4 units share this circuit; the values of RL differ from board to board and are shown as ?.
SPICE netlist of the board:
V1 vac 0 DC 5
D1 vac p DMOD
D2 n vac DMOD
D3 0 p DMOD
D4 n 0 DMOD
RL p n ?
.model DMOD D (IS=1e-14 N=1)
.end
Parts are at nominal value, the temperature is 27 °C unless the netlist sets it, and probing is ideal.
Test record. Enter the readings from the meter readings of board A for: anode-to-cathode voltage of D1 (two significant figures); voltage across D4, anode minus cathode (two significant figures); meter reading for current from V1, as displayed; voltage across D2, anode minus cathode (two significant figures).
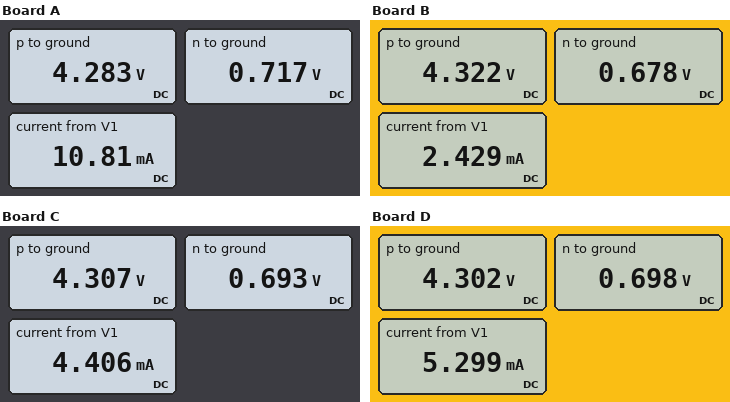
720 mV
720 mV
10.81 mA
-4.3 V
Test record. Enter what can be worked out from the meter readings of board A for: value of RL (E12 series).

330 Ω
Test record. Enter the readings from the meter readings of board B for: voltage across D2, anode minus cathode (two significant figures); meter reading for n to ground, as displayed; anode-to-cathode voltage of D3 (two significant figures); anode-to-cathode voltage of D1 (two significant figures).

-4.3 V
0.678 V
-4.3 V
680 mV
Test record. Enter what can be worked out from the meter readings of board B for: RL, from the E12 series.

1.5 kΩ
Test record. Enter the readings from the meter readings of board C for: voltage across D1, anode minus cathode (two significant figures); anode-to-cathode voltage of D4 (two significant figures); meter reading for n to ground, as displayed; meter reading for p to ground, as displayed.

690 mV
690 mV
0.693 V
4.307 V
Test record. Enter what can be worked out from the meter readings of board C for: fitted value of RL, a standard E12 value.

820 Ω
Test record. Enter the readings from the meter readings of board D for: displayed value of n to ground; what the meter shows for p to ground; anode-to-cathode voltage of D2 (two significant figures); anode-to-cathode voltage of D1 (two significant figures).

0.698 V
4.302 V
-4.3 V
700 mV
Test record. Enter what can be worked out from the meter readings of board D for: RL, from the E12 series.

680 Ω
